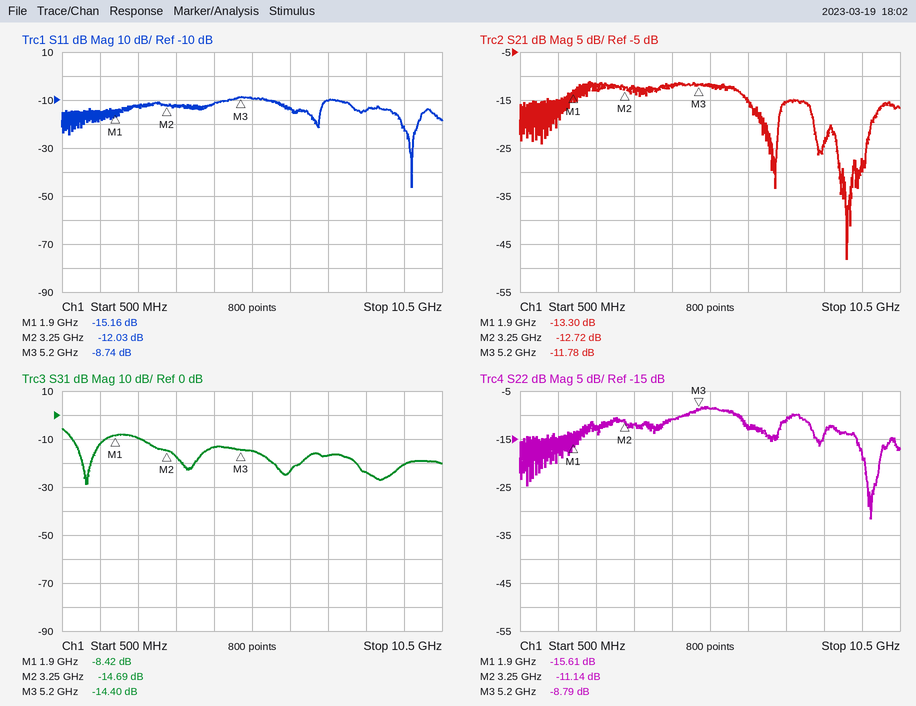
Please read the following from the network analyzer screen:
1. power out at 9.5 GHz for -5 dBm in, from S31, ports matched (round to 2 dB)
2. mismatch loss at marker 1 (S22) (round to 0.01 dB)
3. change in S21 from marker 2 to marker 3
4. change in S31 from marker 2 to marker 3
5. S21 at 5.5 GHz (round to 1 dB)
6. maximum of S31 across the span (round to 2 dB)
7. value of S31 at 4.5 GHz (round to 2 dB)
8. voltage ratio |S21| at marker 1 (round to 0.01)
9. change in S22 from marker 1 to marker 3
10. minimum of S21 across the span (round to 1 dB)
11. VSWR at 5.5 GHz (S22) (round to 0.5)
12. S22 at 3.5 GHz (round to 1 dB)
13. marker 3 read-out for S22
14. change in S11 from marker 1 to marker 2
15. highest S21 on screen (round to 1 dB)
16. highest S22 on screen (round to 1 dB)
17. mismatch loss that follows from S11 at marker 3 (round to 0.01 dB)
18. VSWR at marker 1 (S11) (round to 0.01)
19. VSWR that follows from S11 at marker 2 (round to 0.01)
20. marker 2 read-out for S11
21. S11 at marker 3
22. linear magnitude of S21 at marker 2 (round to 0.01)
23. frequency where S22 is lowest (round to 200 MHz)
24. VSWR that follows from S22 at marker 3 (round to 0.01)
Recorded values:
-26 dBm
0.12 dB
0.94 dB
0.29 dB
-12 dB
-6 dB
-14 dB
0.22
6.82 dB
-48 dB
2.0
-12 dB
-8.79 dB
3.13 dB
-11 dB
-8 dB
0.62 dB
1.42
1.67
-12.03 dB
-8.74 dB
0.23
9.8 GHz
2.14
